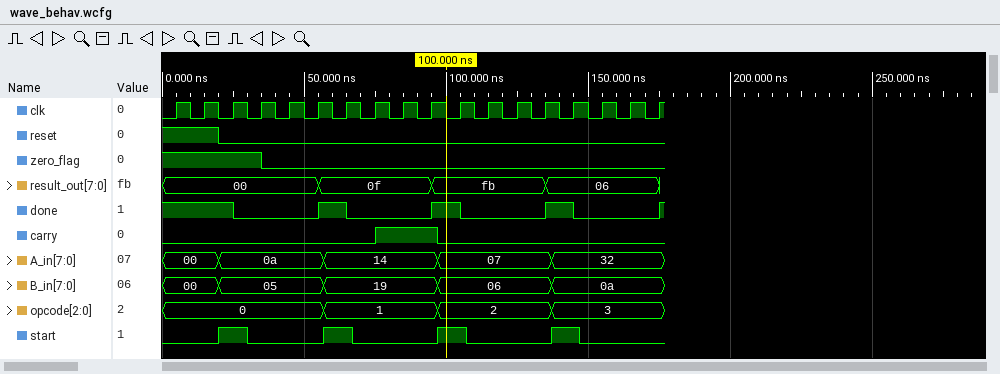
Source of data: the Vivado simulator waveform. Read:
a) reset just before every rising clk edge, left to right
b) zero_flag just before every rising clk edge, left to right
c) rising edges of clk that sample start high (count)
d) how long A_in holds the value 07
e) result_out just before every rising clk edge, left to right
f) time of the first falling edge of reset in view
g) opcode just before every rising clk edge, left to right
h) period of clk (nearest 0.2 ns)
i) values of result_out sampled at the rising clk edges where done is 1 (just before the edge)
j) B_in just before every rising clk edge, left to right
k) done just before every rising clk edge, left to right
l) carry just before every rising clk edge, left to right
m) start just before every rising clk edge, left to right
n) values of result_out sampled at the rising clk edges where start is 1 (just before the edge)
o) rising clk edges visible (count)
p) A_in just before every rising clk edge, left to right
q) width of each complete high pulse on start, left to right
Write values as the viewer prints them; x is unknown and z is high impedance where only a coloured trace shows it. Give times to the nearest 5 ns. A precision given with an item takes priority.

1 1 0 0 0 0 0 0 0 0 0 0 0 0 0 0 0 0
1 1 1 1 0 0 0 0 0 0 0 0 0 0 0 0 0 0
4
40 ns
00, 00, 00, 00, 00, 00, 0f, 0f, 0f, 0f, fb, fb, fb, fb, 06, 06, 06, 06
20 ns
0, 0, 0, 0, 0, 0, 1, 1, 1, 1, 2, 2, 2, 2, 3, 3, 3, 3
10 ns
00, 00, 00, 0f, fb, 06
00, 00, 05, 05, 05, 05, 19, 19, 19, 19, 06, 06, 06, 06, 0a, 0a, 0a, 0a
1 1 1 0 0 0 1 0 0 0 1 0 0 0 1 0 0 0
0 0 0 0 0 0 0 0 1 1 0 0 0 0 0 0 0 0
0 0 1 0 0 0 1 0 0 0 1 0 0 0 1 0 0 0
00, 0f, fb, 06
18
00, 00, 0a, 0a, 0a, 0a, 14, 14, 14, 14, 07, 07, 07, 07, 32, 32, 32, 32
10 ns, 10 ns, 10 ns, 10 ns
